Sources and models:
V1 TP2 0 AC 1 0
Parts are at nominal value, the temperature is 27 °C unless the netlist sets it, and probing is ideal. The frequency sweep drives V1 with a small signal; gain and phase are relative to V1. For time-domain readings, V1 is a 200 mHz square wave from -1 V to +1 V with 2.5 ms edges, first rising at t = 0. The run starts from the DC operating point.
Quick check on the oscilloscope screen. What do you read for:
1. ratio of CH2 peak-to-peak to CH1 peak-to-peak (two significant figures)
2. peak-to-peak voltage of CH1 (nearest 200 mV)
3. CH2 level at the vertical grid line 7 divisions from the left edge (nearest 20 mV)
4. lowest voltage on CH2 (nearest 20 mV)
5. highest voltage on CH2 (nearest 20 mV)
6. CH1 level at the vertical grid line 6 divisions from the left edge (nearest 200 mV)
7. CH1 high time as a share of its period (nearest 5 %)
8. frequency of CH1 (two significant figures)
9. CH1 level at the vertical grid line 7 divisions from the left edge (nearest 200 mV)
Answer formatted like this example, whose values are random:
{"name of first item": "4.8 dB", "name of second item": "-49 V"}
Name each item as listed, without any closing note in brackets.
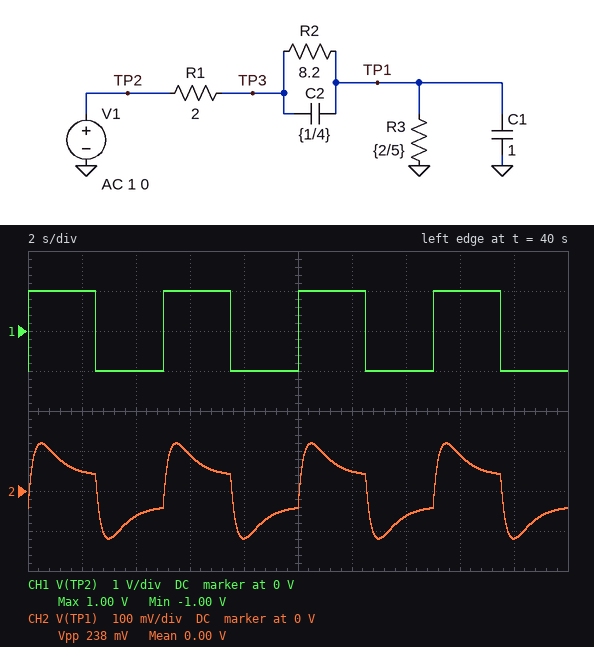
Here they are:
{"ratio of CH2 peak-to-peak to CH1 peak-to-peak": "0.12", "peak-to-peak voltage of CH1": "2.0 V", "CH2 level at the vertical grid line 7 divisions from the left edge": "-60 mV", "lowest voltage on CH2": "-120 mV", "highest voltage on CH2": "120 mV", "CH1 level at the vertical grid line 6 divisions from the left edge": "1.0 V", "CH1 high time as a share of its period": "50 %", "frequency of CH1": "200 mHz", "CH1 level at the vertical grid line 7 divisions from the left edge": "-1.0 V"}
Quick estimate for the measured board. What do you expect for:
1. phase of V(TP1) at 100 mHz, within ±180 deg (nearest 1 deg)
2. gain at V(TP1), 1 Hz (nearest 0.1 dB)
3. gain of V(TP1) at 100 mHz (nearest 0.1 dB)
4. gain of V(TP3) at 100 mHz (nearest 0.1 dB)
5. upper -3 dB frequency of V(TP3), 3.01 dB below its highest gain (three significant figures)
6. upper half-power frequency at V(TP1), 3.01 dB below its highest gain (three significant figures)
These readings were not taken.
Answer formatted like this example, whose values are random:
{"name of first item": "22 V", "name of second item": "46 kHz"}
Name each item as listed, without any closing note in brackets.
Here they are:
{"phase of V(TP1) at 100 mHz, within ±180 deg": "23 deg", "gain at V(TP1), 1 Hz": "-23.6 dB", "gain of V(TP1) at 100 mHz": "-24.9 dB", "gain of V(TP3) at 100 mHz": "-2.1 dB", "upper -3 dB frequency of V(TP3), 3.01 dB below its highest gain": "434 mHz", "upper half-power frequency at V(TP1), 3.01 dB below its highest gain": "1.01 Hz"}
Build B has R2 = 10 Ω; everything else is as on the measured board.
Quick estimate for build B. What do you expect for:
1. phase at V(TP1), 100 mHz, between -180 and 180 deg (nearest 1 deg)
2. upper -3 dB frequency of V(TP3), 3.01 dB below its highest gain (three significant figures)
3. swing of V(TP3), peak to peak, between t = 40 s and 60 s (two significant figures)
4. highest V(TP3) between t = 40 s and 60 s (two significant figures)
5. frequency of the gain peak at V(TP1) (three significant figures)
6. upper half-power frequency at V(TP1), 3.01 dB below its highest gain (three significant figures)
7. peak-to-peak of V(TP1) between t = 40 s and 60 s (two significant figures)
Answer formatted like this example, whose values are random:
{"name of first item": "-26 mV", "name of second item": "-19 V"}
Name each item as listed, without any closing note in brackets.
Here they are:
{"phase at V(TP1), 100 mHz, between -180 and 180 deg": "27 deg", "upper -3 dB frequency of V(TP3), 3.01 dB below its highest gain": "413 mHz", "swing of V(TP3), peak to peak, between t = 40 s and 60 s": "1.7 V", "highest V(TP3) between t = 40 s and 60 s": "830 mV", "frequency of the gain peak at V(TP1)": "384 mHz", "upper half-power frequency at V(TP1), 3.01 dB below its highest gain": "998 mHz", "peak-to-peak of V(TP1) between t = 40 s and 60 s": "250 mV"}
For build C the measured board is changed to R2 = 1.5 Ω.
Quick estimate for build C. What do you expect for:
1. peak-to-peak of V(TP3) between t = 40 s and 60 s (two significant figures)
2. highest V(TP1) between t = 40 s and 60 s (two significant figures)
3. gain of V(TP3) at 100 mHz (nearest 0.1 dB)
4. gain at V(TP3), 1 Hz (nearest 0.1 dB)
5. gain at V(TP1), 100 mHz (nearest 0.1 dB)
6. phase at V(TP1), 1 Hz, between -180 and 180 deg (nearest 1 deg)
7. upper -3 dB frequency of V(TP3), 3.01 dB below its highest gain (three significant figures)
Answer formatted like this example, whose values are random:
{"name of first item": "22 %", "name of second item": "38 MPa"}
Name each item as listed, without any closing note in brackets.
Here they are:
{"peak-to-peak of V(TP3) between t = 40 s and 60 s": "970 mV", "highest V(TP1) between t = 40 s and 60 s": "100 mV", "gain of V(TP3) at 100 mHz": "-6.3 dB", "gain at V(TP3), 1 Hz": "-10.2 dB", "gain at V(TP1), 100 mHz": "-19.9 dB", "phase at V(TP1), 1 Hz, between -180 and 180 deg": "-52 deg", "upper -3 dB frequency of V(TP3), 3.01 dB below its highest gain": "816 mHz"}
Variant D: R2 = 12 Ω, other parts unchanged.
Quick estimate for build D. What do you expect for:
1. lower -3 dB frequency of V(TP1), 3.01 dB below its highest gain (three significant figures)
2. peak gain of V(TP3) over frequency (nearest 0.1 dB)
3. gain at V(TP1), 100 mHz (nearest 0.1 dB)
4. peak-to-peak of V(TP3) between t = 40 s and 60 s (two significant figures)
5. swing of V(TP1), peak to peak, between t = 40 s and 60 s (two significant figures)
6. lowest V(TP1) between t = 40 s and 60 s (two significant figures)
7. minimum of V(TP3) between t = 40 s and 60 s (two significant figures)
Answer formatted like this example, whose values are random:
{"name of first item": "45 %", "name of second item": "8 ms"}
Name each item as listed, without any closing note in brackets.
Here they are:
{"lower -3 dB frequency of V(TP1), 3.01 dB below its highest gain": "140 mHz", "peak gain of V(TP3) over frequency": "-1.3 dB", "gain at V(TP1), 100 mHz": "-25.3 dB", "peak-to-peak of V(TP3) between t = 40 s and 60 s": "1.7 V", "swing of V(TP1), peak to peak, between t = 40 s and 60 s": "250 mV", "lowest V(TP1) between t = 40 s and 60 s": "-130 mV", "minimum of V(TP3) between t = 40 s and 60 s": "-850 mV"}
